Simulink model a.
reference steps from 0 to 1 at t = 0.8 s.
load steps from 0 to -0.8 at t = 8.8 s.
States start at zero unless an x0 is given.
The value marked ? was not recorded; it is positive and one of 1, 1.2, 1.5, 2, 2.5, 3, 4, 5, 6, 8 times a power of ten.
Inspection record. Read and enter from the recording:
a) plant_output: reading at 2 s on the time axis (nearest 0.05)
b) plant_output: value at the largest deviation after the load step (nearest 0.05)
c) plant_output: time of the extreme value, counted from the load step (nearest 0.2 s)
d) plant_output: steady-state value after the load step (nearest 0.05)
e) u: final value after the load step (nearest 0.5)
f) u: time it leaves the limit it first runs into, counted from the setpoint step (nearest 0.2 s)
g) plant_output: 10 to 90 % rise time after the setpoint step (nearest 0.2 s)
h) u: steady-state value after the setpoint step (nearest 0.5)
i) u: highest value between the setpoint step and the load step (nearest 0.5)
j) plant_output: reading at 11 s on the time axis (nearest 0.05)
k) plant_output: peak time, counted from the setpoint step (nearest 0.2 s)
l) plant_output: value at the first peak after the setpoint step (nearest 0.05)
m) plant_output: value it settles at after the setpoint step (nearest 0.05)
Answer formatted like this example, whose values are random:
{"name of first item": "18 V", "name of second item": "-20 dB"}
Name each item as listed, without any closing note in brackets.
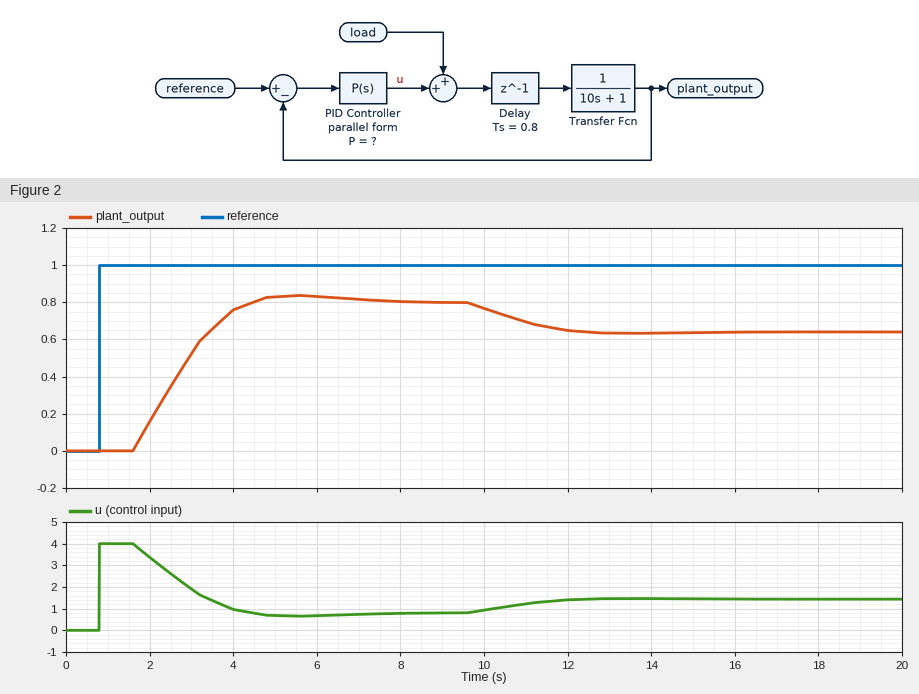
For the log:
{"plant_output: reading at 2 s on the time axis": "0.15", "plant_output: value at the largest deviation after the load step": "0.65", "plant_output: time of the extreme value, counted from the load step": "4.8 s", "plant_output: steady-state value after the load step": "0.65", "u: final value after the load step": "1.5", "u: time it leaves the limit it first runs into, counted from the setpoint step": "0.8 s", "plant_output: 10 to 90 % rise time after the setpoint step": "2.0 s", "u: steady-state value after the setpoint step": "1.0", "u: highest value between the setpoint step and the load step": "4.0", "plant_output: reading at 11 s on the time axis": "0.70", "plant_output: peak time, counted from the setpoint step": "4.8 s", "plant_output: value at the first peak after the setpoint step": "0.85", "plant_output: value it settles at after the setpoint step": "0.80"}
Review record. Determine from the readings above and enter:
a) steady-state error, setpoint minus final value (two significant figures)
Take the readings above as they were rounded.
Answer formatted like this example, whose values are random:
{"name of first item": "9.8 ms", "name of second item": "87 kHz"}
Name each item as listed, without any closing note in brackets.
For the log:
{"steady-state error, setpoint minus final value": "0.20"}
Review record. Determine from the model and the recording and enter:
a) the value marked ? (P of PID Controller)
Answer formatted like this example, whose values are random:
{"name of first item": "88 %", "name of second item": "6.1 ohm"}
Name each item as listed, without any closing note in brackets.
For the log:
{"the value marked ?": "4"}
